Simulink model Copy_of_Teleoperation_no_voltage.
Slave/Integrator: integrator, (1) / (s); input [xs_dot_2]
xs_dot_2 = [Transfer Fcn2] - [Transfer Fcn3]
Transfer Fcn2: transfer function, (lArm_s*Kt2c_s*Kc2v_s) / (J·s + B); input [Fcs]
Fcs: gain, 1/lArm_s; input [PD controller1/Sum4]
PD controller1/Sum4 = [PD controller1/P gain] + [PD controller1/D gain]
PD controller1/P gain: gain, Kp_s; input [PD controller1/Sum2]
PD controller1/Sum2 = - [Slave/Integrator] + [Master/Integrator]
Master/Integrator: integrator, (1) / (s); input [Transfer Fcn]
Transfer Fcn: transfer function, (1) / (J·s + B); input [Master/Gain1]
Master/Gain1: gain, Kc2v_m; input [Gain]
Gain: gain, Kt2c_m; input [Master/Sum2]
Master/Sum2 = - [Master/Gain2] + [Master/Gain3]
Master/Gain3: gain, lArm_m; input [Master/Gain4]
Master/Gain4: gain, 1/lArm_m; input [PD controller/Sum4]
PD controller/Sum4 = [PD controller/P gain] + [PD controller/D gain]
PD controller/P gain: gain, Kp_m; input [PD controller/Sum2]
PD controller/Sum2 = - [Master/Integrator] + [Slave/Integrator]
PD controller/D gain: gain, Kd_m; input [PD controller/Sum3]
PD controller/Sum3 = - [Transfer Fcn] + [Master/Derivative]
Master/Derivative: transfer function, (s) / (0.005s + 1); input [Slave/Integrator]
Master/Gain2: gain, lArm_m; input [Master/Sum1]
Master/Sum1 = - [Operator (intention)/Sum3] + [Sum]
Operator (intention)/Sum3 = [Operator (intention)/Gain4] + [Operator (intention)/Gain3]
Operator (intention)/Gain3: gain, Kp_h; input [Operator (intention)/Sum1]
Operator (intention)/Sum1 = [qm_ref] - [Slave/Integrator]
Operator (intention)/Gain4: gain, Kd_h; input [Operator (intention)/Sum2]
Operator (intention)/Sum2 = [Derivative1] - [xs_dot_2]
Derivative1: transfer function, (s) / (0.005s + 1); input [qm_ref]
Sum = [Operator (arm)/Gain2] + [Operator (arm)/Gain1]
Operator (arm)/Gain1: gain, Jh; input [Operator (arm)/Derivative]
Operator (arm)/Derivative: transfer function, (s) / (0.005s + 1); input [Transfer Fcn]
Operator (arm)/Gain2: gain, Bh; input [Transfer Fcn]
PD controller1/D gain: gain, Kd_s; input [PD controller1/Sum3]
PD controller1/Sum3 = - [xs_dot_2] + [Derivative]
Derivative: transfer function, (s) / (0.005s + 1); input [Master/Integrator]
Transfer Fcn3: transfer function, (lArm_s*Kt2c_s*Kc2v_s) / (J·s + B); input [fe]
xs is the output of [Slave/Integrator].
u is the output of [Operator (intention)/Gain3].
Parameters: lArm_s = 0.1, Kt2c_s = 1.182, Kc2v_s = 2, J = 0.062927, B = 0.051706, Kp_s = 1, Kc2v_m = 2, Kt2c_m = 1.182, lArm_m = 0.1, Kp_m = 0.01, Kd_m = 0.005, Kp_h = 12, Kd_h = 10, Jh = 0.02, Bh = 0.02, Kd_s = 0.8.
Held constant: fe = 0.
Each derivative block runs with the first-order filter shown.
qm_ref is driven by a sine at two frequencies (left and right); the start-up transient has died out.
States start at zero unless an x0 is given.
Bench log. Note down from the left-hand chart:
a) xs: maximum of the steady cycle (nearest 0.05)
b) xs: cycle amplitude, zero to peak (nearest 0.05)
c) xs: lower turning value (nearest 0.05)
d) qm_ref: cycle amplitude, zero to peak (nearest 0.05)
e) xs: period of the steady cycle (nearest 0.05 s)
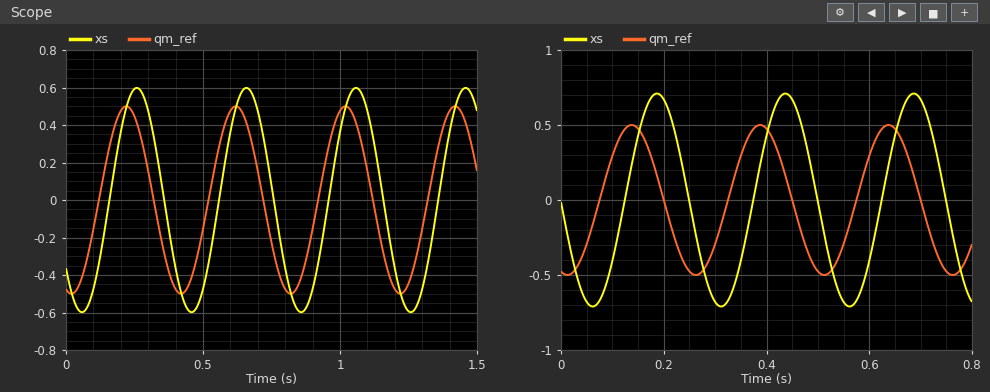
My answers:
0.60
0.60
-0.60
0.50
0.40 s
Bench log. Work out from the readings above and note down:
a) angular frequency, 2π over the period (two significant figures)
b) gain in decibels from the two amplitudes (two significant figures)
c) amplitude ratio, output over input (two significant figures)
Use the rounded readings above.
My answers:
16 rad/s
1.6 dB
1.2
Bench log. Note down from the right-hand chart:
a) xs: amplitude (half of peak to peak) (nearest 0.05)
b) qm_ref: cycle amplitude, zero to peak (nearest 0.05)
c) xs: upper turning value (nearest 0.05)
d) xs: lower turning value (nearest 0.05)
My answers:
0.70
0.50
0.70
-0.70
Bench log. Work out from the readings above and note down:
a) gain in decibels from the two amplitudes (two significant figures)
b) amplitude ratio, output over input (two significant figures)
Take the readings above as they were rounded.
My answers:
2.9 dB
1.4
